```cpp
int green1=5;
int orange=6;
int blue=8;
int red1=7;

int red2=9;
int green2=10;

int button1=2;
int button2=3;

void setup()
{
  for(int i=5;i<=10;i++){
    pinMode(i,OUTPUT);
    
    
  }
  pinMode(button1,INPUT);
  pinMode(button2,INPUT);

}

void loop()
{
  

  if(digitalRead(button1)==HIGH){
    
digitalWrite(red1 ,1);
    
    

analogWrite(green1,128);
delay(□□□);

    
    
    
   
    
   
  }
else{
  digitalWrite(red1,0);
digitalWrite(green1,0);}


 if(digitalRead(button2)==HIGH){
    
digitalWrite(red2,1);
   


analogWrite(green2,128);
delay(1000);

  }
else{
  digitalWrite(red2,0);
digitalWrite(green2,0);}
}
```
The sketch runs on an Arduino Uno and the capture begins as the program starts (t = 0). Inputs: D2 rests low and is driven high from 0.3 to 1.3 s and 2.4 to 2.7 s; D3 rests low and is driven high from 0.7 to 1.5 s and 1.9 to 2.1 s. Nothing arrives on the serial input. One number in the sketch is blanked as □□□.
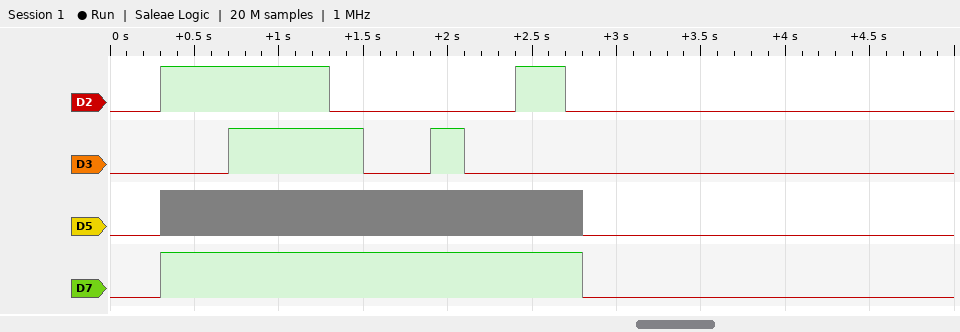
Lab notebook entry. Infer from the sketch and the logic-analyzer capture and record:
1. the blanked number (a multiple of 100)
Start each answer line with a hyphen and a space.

- 2500
